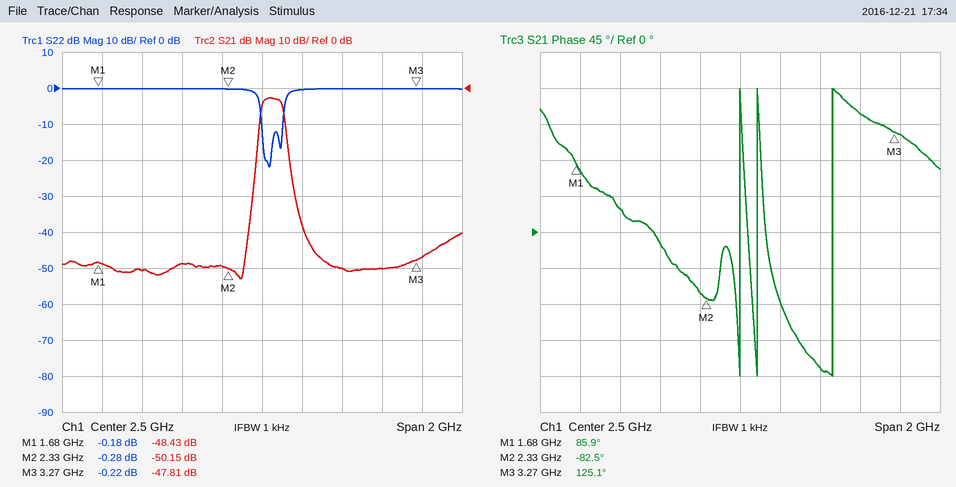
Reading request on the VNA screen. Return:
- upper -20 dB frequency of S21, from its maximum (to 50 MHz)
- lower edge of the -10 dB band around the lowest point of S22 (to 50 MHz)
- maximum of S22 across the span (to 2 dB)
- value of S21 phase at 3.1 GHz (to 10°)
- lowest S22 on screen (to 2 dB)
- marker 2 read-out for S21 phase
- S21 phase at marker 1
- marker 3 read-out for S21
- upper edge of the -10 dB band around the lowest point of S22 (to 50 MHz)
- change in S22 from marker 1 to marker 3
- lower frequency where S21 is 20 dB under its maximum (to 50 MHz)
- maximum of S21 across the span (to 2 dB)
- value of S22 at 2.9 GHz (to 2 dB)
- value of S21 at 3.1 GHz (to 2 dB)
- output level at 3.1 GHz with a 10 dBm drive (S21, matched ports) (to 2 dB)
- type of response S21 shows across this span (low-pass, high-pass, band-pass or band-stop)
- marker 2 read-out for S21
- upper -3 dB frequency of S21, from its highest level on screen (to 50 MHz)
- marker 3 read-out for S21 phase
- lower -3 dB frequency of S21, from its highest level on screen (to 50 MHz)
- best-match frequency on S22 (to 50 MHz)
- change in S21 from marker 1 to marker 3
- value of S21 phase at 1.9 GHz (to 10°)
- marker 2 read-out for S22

2.65 GHz
2.50 GHz
0 dB
150°
-22 dB
-82.5°
85.9°
-47.81 dB
2.60 GHz
-0.04 dB
2.45 GHz
-2 dB
0 dB
-50 dB
-40 dBm
band-pass
-50.15 dB
2.60 GHz
125.1°
2.50 GHz
2.55 GHz
0.62 dB
30°
-0.28 dB
